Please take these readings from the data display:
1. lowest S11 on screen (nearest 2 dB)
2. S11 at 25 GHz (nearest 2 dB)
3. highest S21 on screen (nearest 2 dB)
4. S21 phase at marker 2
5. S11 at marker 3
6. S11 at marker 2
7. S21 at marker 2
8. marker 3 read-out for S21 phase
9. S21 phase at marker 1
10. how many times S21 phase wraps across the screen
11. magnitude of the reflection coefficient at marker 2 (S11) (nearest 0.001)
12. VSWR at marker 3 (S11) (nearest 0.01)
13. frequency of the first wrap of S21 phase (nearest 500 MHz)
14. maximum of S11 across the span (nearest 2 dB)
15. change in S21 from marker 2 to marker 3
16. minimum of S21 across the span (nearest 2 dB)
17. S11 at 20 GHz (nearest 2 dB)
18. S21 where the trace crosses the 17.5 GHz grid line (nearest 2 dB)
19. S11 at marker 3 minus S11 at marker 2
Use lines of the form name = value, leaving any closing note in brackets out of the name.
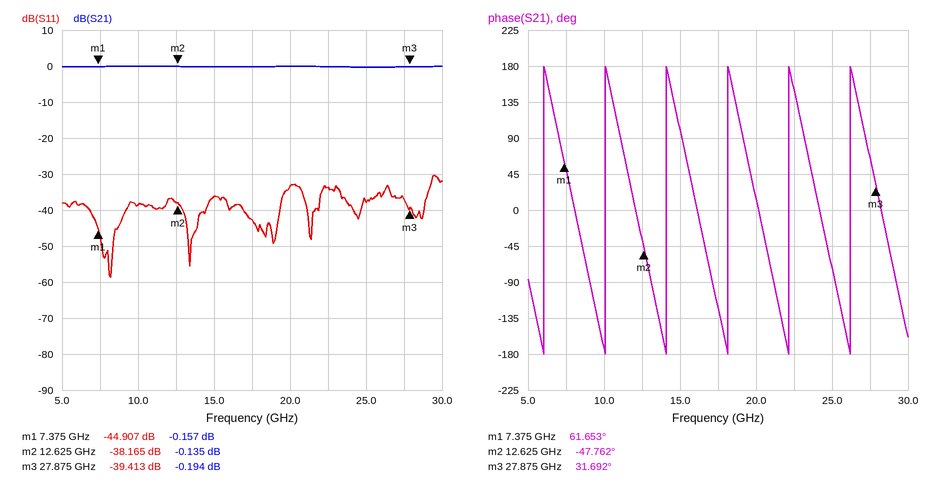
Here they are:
lowest S11 on screen = -58 dB
S11 at 25 GHz = -38 dB
highest S21 on screen = 0 dB
S21 phase at marker 2 = -47.762°
S11 at marker 3 = -39.413 dB
S11 at marker 2 = -38.165 dB
S21 at marker 2 = -0.135 dB
marker 3 read-out for S21 phase = 31.692°
S21 phase at marker 1 = 61.653°
how many times S21 phase wraps across the screen = 6
magnitude of the reflection coefficient at marker 2 (S11) = 0.012
VSWR at marker 3 (S11) = 1.02
frequency of the first wrap of S21 phase = 6.0 GHz
maximum of S11 across the span = -30 dB
change in S21 from marker 2 to marker 3 = -0.059 dB
minimum of S21 across the span = 0 dB
S11 at 20 GHz = -34 dB
S21 where the trace crosses the 17.5 GHz grid line = 0 dB
S11 at marker 3 minus S11 at marker 2 = -1.248 dB
